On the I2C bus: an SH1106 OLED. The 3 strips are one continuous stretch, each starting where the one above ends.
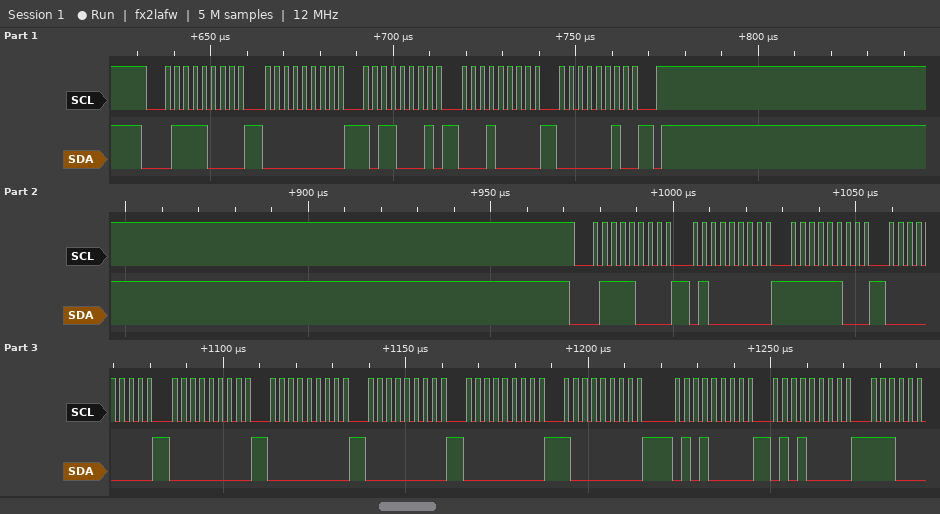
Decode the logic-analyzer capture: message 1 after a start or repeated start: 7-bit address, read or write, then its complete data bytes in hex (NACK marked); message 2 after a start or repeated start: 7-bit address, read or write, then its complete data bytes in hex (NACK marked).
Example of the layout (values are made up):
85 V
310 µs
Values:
0x3C write: 00 B1 10 02
0x3C write: 40 FC 00 00 00 00 00 80 50 50
